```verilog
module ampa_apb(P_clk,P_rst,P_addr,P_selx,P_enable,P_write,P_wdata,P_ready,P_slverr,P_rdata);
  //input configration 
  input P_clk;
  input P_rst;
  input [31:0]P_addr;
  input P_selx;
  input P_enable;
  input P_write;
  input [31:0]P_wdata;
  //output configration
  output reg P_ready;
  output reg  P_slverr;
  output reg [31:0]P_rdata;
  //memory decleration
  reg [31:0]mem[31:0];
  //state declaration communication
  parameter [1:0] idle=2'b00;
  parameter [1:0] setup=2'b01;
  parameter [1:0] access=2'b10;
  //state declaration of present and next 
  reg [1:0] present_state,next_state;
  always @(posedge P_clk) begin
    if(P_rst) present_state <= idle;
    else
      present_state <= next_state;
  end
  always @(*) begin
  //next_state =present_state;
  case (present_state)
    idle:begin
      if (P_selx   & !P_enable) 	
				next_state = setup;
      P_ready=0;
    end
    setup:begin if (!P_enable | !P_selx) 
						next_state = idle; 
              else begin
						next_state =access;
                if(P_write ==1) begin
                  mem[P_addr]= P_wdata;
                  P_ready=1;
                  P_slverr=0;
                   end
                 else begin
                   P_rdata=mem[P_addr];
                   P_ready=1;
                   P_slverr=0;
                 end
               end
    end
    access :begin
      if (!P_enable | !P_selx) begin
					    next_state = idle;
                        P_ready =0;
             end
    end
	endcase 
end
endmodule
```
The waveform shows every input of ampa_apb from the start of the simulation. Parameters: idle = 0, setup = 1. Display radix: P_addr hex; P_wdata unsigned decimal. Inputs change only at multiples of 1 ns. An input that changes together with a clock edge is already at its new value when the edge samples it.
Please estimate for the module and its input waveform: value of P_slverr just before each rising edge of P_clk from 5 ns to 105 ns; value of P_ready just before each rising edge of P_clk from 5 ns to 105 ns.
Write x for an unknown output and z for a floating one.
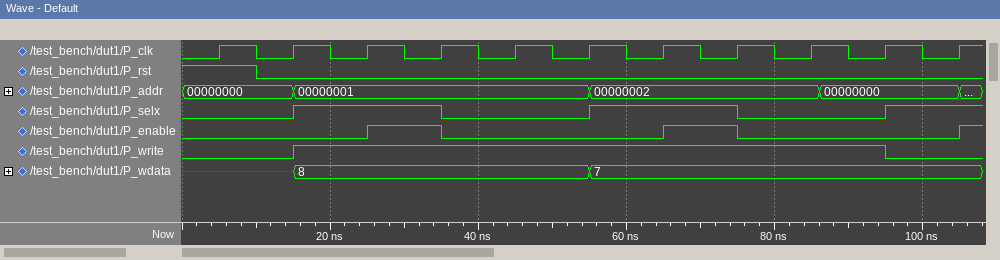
x x x 0 0 0 0 0 0 0 0
x 0 0 1 0 0 0 1 0 0 0
